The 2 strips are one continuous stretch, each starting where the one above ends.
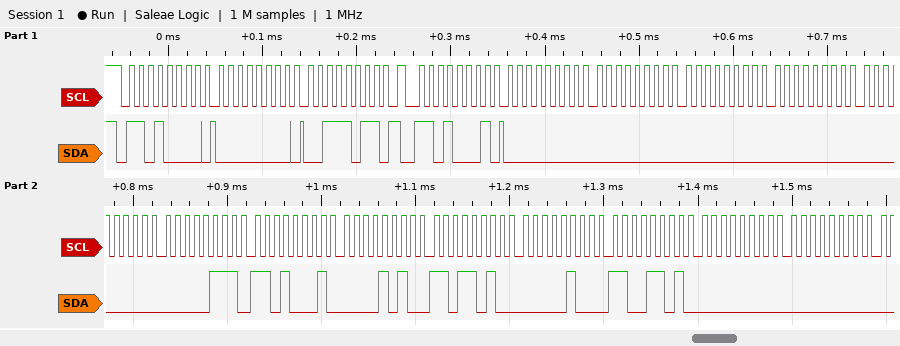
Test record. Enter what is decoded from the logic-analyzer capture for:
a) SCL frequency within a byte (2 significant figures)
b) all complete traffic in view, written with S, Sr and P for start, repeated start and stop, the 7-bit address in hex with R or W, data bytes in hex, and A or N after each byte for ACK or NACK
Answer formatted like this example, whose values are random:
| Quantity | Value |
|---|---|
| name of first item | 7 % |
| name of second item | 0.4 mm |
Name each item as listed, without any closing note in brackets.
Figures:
| Quantity | Value |
|---|---|
| SCL frequency within a byte | 100 kHz |
| all complete traffic in view, written with S, Sr and P for start, repeated start and stop, the 7-bit address in hex with R or W, data bytes in hex, and A or N after each byte for ACK or NACK | S 68W A 00 A 3B A Sr 68R A 00 A 00 A 00 A 00 A 00 A 07 A D1 A 0A A DA A 04 A CD A 00 A 00 A |
